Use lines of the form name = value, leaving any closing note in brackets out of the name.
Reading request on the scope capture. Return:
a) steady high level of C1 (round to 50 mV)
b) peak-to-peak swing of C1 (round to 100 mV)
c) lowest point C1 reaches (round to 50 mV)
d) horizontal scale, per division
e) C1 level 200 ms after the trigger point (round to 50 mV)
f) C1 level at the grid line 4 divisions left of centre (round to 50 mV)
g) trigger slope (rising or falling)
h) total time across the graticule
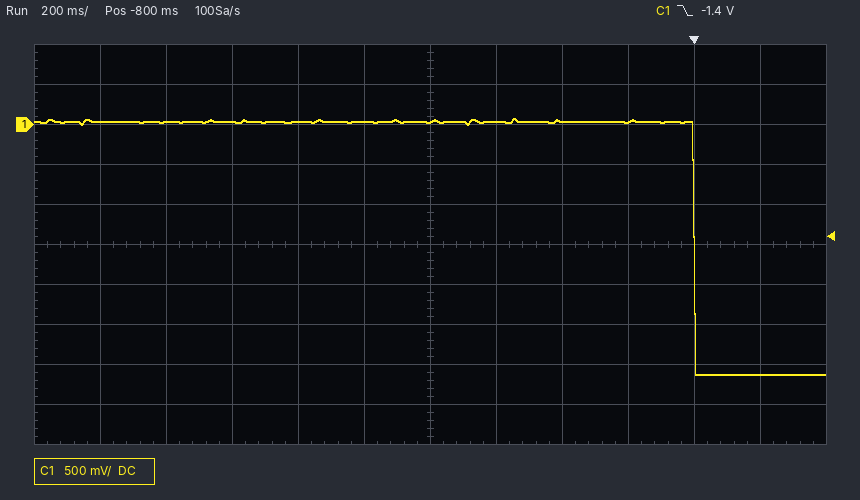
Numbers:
steady high level of C1 = 50 mV
peak-to-peak swing of C1 = 3.20 V
lowest point C1 reaches = -3.10 V
horizontal scale, per division = 200 ms
C1 level 200 ms after the trigger point = -3.10 V
C1 level at the grid line 4 divisions left of centre = 50 mV
trigger slope = falling
total time across the graticule = 2.4 s
